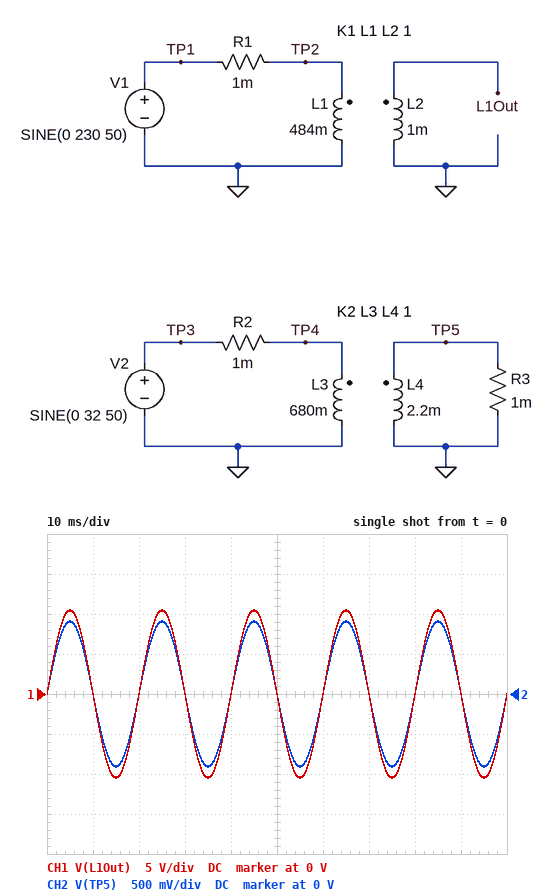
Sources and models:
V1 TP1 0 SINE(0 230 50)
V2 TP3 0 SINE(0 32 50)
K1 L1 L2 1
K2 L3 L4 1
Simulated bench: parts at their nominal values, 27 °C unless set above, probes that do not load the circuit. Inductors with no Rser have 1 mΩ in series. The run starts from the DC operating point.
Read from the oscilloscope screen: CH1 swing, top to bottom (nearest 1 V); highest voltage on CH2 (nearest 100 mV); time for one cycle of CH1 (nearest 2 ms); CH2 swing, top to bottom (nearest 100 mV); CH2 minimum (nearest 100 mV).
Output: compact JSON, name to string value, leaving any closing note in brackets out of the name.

{"CH1 swing, top to bottom": "21 V", "highest voltage on CH2": "900 mV", "time for one cycle of CH1": "20 ms", "CH2 swing, top to bottom": "1.8 V", "CH2 minimum": "-900 mV"}
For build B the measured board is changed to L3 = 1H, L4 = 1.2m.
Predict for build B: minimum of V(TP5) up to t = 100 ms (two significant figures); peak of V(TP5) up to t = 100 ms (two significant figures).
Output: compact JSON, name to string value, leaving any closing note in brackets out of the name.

{"minimum of V(TP5) up to t = 100 ms": "-550 mV", "peak of V(TP5) up to t = 100 ms": "550 mV"}
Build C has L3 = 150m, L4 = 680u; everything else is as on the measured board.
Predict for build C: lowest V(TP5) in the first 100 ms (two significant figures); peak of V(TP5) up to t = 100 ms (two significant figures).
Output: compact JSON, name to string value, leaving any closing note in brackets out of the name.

{"lowest V(TP5) in the first 100 ms": "-1.1 V", "peak of V(TP5) up to t = 100 ms": "1.1 V"}
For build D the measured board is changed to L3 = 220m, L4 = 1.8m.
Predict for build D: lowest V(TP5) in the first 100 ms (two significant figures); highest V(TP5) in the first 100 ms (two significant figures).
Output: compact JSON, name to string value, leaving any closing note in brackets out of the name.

{"lowest V(TP5) in the first 100 ms": "-1.4 V", "highest V(TP5) in the first 100 ms": "1.4 V"}
